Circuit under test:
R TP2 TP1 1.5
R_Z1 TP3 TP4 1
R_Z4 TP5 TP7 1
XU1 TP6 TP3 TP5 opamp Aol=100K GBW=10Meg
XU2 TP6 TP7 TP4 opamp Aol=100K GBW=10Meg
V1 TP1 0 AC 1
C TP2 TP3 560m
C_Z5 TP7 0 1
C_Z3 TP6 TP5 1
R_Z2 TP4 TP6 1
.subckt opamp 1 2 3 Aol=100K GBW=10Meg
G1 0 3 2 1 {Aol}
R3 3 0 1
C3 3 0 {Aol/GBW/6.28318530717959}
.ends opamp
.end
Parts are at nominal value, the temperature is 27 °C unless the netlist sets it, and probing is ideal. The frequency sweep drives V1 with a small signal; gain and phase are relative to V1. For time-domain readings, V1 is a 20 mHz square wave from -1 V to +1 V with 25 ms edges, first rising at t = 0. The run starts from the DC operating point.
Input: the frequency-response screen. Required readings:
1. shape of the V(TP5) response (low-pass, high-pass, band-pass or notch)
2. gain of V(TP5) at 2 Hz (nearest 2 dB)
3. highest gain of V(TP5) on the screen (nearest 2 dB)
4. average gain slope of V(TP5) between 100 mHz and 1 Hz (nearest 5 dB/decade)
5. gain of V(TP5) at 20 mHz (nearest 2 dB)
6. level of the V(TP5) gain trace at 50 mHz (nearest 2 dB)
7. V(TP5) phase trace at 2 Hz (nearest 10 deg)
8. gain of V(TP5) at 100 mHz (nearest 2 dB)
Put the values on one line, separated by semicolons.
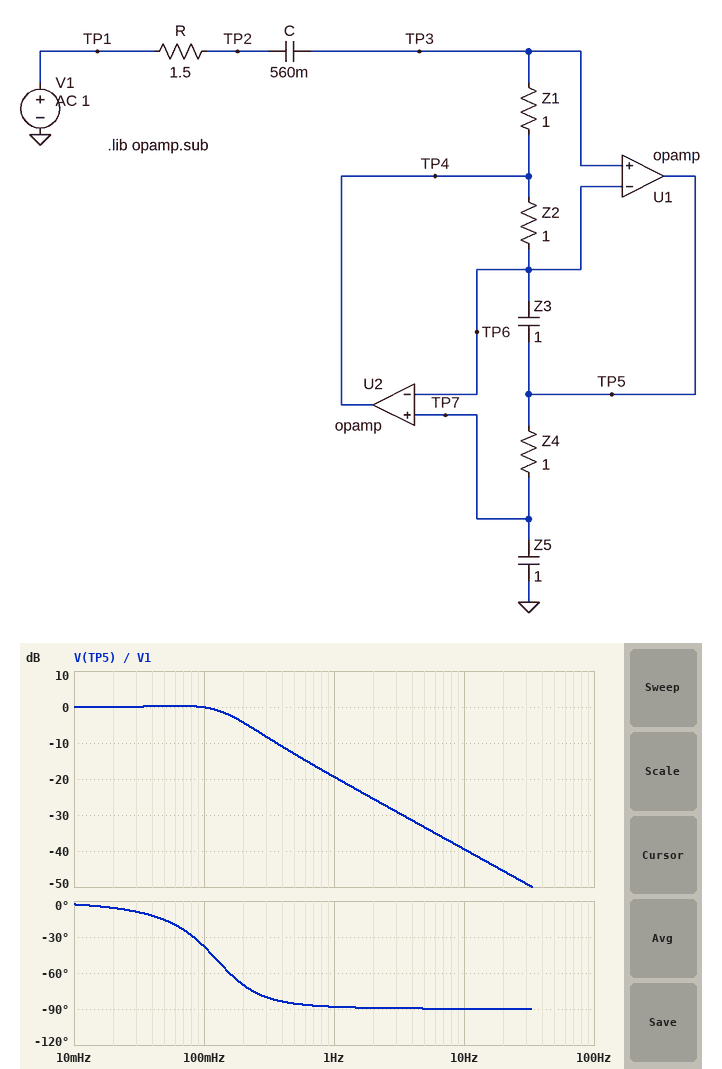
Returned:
low-pass; -26 dB; 0 dB; -20 dB/decade; 0 dB; 0 dB; -90 deg; 0 dB
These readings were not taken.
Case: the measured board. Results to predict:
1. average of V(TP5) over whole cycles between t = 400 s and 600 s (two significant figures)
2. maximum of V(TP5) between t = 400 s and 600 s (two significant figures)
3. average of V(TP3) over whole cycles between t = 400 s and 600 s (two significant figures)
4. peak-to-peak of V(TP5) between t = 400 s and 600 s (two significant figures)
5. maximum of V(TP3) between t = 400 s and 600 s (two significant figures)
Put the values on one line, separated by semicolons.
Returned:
990 mV; 2.1 V; 990 mV; 2.3 V; 2.1 V
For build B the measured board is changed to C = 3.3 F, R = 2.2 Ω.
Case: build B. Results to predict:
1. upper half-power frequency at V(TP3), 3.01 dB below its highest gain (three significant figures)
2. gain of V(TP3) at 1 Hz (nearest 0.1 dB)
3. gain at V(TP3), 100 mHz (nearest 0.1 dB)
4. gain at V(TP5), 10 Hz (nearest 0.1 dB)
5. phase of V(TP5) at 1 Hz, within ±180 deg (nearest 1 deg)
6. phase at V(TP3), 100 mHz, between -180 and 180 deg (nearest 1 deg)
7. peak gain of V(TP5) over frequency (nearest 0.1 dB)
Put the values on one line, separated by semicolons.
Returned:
117 mHz; -38.7 dB; 12.7 dB; -42.8 dB; -98 deg; -55 deg; 15.4 dB
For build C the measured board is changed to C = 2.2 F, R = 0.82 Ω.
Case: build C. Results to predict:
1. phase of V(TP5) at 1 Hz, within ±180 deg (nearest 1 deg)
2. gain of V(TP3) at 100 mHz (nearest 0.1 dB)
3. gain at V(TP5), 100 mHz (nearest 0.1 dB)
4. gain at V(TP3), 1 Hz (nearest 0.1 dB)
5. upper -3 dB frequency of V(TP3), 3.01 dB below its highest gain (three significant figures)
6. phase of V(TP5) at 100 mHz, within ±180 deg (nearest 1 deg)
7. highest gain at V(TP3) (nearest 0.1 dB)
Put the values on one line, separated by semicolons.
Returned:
-94 deg; 2.7 dB; 4.1 dB; -30.0 dB; 205 mHz; 9 deg; 6.3 dB
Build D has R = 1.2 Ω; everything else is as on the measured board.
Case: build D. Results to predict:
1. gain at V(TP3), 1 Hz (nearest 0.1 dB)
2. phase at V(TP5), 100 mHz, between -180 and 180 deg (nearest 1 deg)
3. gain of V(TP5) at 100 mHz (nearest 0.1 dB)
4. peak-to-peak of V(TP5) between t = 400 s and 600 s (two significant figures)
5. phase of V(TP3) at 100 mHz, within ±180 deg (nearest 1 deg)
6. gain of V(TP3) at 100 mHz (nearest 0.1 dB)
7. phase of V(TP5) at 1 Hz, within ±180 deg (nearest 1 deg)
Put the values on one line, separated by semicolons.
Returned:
-33.6 dB; -33 deg; -0.4 dB; 2.1 V; -65 deg; -1.9 dB; -85 deg
